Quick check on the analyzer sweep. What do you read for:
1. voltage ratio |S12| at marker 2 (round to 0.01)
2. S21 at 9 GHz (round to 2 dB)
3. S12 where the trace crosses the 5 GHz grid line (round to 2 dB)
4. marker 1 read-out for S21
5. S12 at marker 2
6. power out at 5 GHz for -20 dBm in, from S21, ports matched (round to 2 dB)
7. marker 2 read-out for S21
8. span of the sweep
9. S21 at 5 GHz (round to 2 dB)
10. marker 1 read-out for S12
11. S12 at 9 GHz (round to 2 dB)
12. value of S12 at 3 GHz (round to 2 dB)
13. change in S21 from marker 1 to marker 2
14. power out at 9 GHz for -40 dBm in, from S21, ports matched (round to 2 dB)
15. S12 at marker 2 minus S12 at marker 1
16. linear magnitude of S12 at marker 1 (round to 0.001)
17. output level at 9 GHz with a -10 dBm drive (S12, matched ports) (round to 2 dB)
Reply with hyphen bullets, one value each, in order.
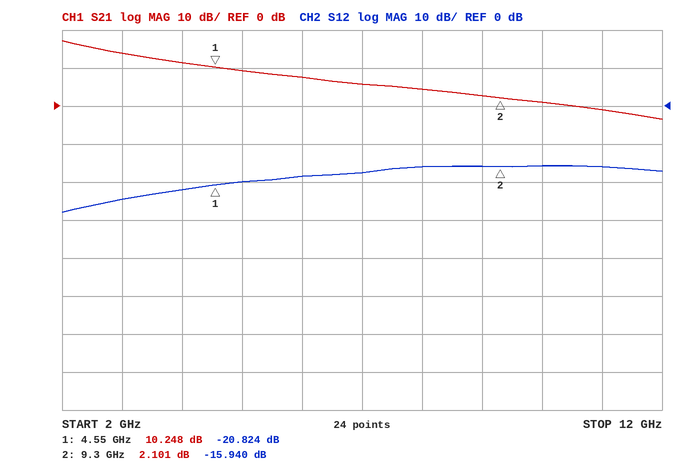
- 0.16
- 2 dB
- -20 dB
- 10.248 dB
- -15.940 dB
- -10 dBm
- 2.101 dB
- 10 GHz
- 10 dB
- -20.824 dB
- -16 dB
- -24 dB
- -8.147 dB
- -38 dBm
- 4.884 dB
- 0.091
- -26 dBm
